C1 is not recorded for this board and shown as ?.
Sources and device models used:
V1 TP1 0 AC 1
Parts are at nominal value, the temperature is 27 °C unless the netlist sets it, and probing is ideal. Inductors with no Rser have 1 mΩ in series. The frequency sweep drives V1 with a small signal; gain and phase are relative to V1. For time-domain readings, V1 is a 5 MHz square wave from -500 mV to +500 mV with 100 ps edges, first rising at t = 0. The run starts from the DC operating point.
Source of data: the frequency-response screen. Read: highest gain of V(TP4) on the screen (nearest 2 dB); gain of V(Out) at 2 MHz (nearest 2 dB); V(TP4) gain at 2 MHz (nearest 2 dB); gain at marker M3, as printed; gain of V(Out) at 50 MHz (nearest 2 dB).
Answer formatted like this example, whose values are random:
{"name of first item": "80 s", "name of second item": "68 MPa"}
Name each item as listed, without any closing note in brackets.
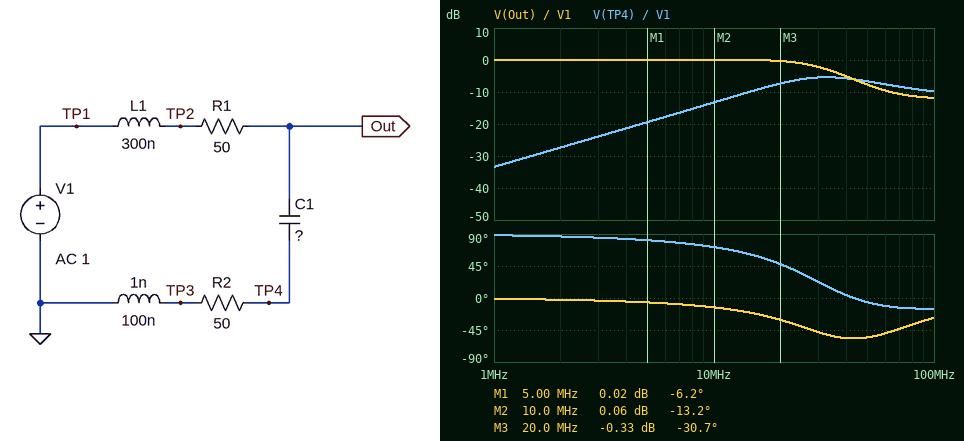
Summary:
{"highest gain of V(TP4) on the screen": "-6 dB", "gain of V(Out) at 2 MHz": "0 dB", "V(TP4) gain at 2 MHz": "-28 dB", "gain at marker M3, as printed": "-0.33 dB", "gain of V(Out) at 50 MHz": "-8 dB"}
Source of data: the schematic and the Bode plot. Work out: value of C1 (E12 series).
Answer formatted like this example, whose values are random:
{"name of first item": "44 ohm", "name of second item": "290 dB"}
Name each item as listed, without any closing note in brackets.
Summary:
{"value of C1": "68 pF"}
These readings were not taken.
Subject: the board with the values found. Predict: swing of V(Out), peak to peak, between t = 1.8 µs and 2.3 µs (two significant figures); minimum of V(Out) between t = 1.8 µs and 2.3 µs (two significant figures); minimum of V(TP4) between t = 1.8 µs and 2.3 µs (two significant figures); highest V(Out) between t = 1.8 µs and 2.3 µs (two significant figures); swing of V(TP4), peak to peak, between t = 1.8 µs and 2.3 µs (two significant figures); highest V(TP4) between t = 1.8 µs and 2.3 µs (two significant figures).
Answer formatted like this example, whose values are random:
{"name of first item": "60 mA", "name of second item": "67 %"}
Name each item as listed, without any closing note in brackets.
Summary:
{"swing of V(Out), peak to peak, between t = 1.8 µs and 2.3 µs": "1.1 V", "minimum of V(Out) between t = 1.8 µs and 2.3 µs": "-560 mV", "minimum of V(TP4) between t = 1.8 µs and 2.3 µs": "-340 mV", "highest V(Out) between t = 1.8 µs and 2.3 µs": "560 mV", "swing of V(TP4), peak to peak, between t = 1.8 µs and 2.3 µs": "690 mV", "highest V(TP4) between t = 1.8 µs and 2.3 µs": "340 mV"}
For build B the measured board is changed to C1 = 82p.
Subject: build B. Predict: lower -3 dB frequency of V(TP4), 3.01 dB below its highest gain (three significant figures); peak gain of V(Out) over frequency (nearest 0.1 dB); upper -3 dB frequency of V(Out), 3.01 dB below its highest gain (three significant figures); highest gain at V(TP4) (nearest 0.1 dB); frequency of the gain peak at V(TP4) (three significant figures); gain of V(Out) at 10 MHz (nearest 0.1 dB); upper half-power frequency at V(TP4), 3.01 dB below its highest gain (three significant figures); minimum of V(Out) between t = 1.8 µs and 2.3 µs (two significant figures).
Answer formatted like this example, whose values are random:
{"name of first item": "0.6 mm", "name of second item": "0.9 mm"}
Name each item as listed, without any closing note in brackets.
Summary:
{"lower -3 dB frequency of V(TP4), 3.01 dB below its highest gain": "15.0 MHz", "peak gain of V(Out) over frequency": "0 dB", "upper -3 dB frequency of V(Out), 3.01 dB below its highest gain": "28.5 MHz", "highest gain at V(TP4)": "-5.5 dB", "frequency of the gain peak at V(TP4)": "29.6 MHz", "gain of V(Out) at 10 MHz": "-0.1 dB", "upper half-power frequency at V(TP4), 3.01 dB below its highest gain": "68.8 MHz", "minimum of V(Out) between t = 1.8 µs and 2.3 µs": "-540 mV"}
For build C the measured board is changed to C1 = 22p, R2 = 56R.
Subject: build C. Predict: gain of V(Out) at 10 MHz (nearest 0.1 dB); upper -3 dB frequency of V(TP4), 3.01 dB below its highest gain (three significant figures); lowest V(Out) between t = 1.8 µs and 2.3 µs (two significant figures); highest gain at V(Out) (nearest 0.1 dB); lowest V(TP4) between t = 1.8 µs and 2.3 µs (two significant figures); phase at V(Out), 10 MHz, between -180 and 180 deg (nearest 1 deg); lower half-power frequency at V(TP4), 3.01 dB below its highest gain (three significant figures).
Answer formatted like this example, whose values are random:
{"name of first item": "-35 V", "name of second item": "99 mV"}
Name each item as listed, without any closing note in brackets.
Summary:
{"gain of V(Out) at 10 MHz": "0.2 dB", "upper -3 dB frequency of V(TP4), 3.01 dB below its highest gain": "90.7 MHz", "lowest V(Out) between t = 1.8 µs and 2.3 µs": "-710 mV", "highest gain at V(Out)": "1.9 dB", "lowest V(TP4) between t = 1.8 µs and 2.3 µs": "-310 mV", "phase at V(Out), 10 MHz, between -180 and 180 deg": "-4 deg", "lower half-power frequency at V(TP4), 3.01 dB below its highest gain": "38.6 MHz"}
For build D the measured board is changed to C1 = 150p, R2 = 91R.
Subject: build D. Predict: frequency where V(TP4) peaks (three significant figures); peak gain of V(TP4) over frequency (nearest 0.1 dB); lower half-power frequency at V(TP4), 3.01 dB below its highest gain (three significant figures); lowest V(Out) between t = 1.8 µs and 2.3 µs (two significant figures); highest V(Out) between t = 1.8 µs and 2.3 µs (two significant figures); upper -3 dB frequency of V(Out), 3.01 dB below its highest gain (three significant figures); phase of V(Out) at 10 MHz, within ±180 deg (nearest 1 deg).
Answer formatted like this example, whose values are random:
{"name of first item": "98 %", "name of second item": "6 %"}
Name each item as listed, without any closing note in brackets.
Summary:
{"frequency where V(TP4) peaks": "21.4 MHz", "peak gain of V(TP4) over frequency": "-3.7 dB", "lower half-power frequency at V(TP4), 3.01 dB below its highest gain": "6.82 MHz", "lowest V(Out) between t = 1.8 µs and 2.3 µs": "-500 mV", "highest V(Out) between t = 1.8 µs and 2.3 µs": "500 mV", "upper -3 dB frequency of V(Out), 3.01 dB below its highest gain": "19.9 MHz", "phase of V(Out) at 10 MHz, within ±180 deg": "-18 deg"}
